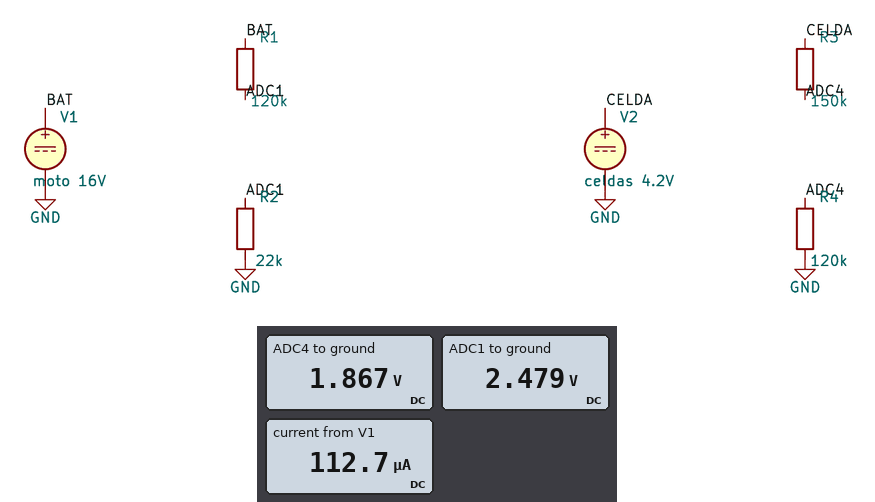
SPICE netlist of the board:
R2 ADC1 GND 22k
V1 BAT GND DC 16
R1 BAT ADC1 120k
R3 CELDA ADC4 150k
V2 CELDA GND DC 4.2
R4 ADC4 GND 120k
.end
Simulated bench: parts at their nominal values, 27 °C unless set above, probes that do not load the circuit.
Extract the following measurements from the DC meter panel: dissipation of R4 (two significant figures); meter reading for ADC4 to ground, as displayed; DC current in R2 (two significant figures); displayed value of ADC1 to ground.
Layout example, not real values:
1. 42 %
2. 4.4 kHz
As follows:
1. 29 µW
2. 1.867 V
3. 110 µA
4. 2.479 V
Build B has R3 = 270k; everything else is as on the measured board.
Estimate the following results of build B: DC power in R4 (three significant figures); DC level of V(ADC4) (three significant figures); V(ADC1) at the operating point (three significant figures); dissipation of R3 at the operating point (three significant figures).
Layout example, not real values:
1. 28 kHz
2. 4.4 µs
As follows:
1. 13.9 µW
2. 1.29 V
3. 2.48 V
4. 31.3 µW
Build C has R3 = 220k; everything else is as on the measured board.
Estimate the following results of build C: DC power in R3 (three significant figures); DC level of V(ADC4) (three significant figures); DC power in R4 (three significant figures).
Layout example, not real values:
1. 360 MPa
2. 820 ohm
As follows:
1. 33.6 µW
2. 1.48 V
3. 18.3 µW
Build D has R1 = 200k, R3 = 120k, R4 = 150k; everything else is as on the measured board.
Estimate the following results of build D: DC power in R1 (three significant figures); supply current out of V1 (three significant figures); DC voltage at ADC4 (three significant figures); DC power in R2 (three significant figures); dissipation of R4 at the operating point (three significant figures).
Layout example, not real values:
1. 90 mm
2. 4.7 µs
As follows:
1. 1.04 mW
2. 72.1 µA
3. 2.33 V
4. 114 µW
5. 36.3 µW
